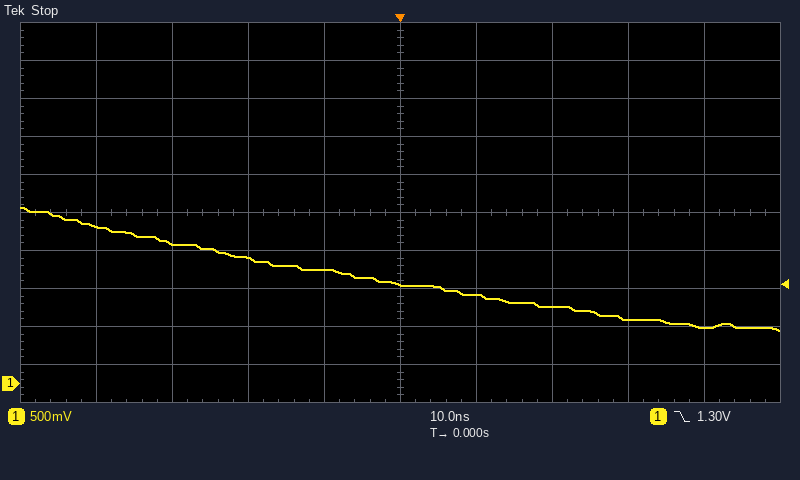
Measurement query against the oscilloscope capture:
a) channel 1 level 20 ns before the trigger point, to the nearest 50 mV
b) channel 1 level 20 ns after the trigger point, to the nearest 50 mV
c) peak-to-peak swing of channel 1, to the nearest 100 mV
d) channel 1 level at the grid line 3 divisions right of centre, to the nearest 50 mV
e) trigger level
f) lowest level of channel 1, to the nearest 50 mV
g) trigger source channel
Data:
1.65 V
1.00 V
1.60 V
850 mV
1.30 V
700 mV
channel 1
